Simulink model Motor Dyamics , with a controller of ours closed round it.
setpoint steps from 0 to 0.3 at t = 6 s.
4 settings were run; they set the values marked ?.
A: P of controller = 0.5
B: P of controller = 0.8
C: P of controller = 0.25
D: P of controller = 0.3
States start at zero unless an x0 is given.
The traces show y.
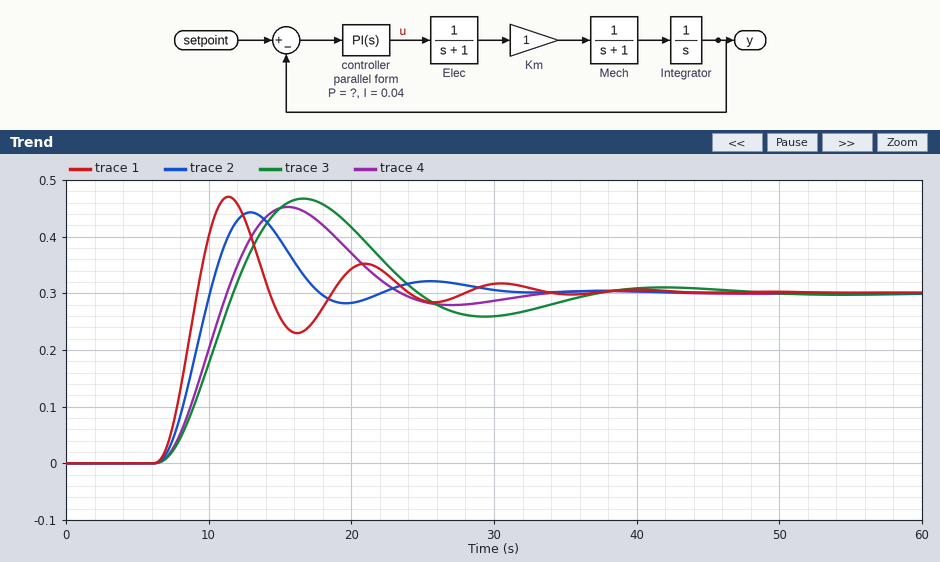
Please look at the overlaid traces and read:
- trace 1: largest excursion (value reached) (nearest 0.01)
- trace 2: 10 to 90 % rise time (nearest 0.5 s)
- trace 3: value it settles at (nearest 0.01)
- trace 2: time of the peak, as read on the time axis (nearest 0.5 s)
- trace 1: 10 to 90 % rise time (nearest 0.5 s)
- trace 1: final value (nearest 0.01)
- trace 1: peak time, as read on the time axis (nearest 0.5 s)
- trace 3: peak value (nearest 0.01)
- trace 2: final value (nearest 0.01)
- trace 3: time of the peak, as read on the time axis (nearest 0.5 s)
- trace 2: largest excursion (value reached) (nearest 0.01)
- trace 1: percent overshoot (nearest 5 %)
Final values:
0.47
2.5 s
0.30
13.0 s
2.0 s
0.30
11.5 s
0.47
0.30
16.5 s
0.44
55 %
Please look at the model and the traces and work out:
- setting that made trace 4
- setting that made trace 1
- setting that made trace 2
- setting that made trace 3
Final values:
D
B
A
C
